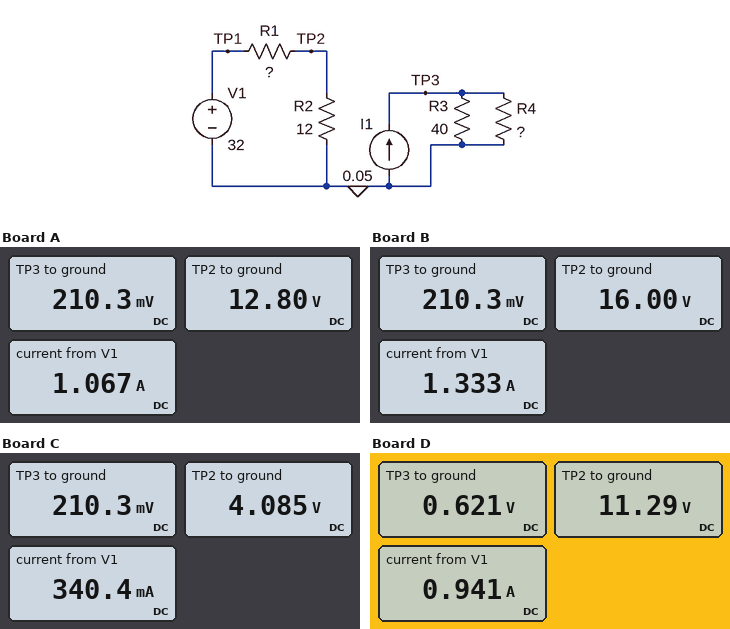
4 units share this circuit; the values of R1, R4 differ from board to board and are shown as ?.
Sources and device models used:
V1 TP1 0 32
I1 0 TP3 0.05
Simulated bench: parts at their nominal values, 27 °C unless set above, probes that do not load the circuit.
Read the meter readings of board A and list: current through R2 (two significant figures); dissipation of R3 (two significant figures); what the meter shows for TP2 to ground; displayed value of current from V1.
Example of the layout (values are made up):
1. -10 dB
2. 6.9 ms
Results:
1. 1.1 A
2. 1.1 mW
3. 12.80 V
4. 1.067 A
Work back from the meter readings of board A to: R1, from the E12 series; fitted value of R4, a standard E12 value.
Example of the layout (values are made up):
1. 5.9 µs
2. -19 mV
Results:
1. 18 Ω
2. 4.7 Ω
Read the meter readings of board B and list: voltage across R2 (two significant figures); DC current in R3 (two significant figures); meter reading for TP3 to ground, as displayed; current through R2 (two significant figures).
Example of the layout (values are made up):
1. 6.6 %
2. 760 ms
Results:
1. 16 V
2. 5.3 mA
3. 210.3 mV
4. 1.3 A
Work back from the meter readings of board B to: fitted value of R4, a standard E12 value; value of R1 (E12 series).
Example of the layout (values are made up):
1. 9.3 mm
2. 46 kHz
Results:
1. 4.7 Ω
2. 12 Ω
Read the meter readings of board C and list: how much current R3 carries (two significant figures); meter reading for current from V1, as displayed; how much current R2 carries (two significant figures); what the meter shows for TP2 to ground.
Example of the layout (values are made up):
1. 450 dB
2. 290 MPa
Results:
1. 5.3 mA
2. 340.4 mA
3. 340 mA
4. 4.085 V
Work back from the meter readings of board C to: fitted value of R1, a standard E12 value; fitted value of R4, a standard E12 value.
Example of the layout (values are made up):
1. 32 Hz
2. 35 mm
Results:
1. 82 Ω
2. 4.7 Ω
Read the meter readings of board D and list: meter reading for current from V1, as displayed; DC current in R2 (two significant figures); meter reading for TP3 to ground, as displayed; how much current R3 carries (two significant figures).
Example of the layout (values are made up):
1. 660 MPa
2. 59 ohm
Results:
1. 0.941 A
2. 940 mA
3. 0.621 V
4. 16 mA
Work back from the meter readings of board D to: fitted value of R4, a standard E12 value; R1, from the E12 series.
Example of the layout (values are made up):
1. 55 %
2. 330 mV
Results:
1. 18 Ω
2. 22 Ω
